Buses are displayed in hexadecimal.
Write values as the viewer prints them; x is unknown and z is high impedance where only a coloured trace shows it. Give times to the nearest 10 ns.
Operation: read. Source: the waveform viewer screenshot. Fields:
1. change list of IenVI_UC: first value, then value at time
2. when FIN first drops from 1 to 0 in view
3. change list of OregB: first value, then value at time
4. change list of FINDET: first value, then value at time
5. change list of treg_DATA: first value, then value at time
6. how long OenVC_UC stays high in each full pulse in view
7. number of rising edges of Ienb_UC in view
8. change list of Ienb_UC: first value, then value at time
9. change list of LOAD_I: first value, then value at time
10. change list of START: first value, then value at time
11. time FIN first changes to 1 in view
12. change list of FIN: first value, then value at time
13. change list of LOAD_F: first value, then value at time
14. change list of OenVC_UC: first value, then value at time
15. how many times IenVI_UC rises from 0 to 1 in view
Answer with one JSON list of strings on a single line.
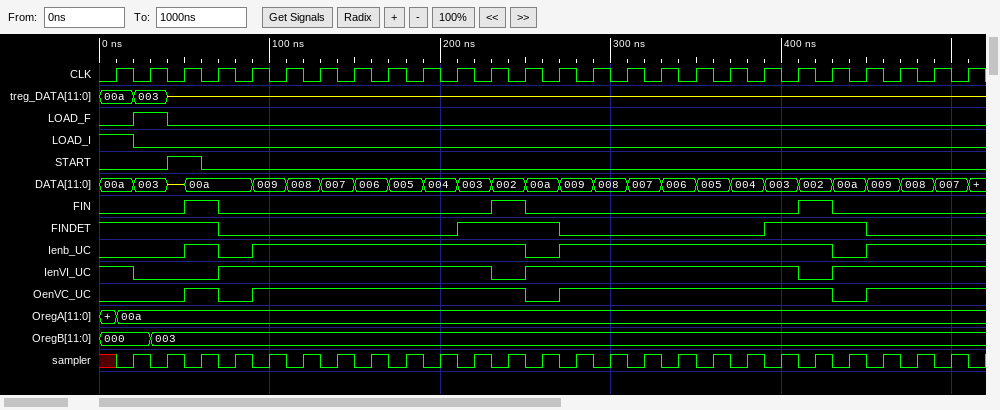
["1, 0 at 20 ns, 1 at 70 ns, 0 at 230 ns, 1 at 250 ns, 0 at 410 ns, 1 at 430 ns", "70 ns", "000, 003 at 30 ns", "1, 0 at 70 ns, 1 at 210 ns, 0 at 270 ns, 1 at 390 ns, 0 at 450 ns", "00a, 003 at 20 ns, z at 40 ns", "20 ns, 160 ns, 160 ns", "4", "0, 1 at 50 ns, 0 at 70 ns, 1 at 90 ns, 0 at 250 ns, 1 at 270 ns, 0 at 430 ns, 1 at 450 ns", "1, 0 at 20 ns", "0, 1 at 40 ns, 0 at 60 ns", "50 ns", "0, 1 at 50 ns, 0 at 70 ns, 1 at 230 ns, 0 at 250 ns, 1 at 410 ns, 0 at 430 ns", "0, 1 at 20 ns, 0 at 40 ns", "0, 1 at 50 ns, 0 at 70 ns, 1 at 90 ns, 0 at 250 ns, 1 at 270 ns, 0 at 430 ns, 1 at 450 ns", "3"]
